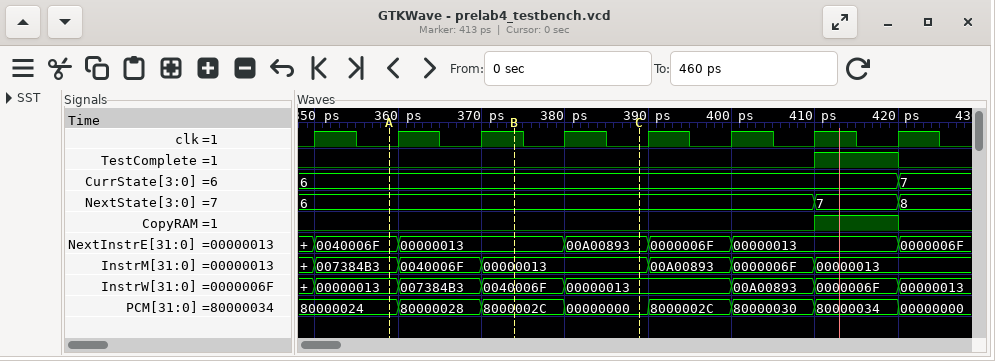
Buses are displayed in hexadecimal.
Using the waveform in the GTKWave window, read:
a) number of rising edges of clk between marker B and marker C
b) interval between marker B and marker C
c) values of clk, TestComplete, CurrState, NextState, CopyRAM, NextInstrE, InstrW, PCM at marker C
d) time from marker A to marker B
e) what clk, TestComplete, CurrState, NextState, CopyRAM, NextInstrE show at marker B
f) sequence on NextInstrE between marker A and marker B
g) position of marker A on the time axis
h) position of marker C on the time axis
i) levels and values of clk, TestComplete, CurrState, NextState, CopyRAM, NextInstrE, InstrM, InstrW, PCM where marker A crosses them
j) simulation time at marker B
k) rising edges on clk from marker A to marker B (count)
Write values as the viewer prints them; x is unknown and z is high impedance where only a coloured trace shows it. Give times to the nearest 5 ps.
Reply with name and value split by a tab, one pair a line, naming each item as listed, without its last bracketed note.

number of rising edges of clk between marker B and marker C	1
interval between marker B and marker C	15 ps
values of clk, TestComplete, CurrState, NextState, CopyRAM, NextInstrE, InstrW, PCM at marker C	clk=0, TestComplete=0, CurrState=6, NextState=6, CopyRAM=0, NextInstrE=00A00893, InstrW=00000013, PCM=00000000
time from marker A to marker B	15 ps
what clk, TestComplete, CurrState, NextState, CopyRAM, NextInstrE show at marker B	clk=1, TestComplete=0, CurrState=6, NextState=6, CopyRAM=0, NextInstrE=00000013
sequence on NextInstrE between marker A and marker B	0040006F, 00000013
position of marker A on the time axis	360 ps
position of marker C on the time axis	390 ps
levels and values of clk, TestComplete, CurrState, NextState, CopyRAM, NextInstrE, InstrM, InstrW, PCM where marker A crosses them	clk=0, TestComplete=0, CurrState=6, NextState=6, CopyRAM=0, NextInstrE=0040006F, InstrM=007384B3, InstrW=00000013, PCM=80000024
simulation time at marker B	375 ps
rising edges on clk from marker A to marker B	2
